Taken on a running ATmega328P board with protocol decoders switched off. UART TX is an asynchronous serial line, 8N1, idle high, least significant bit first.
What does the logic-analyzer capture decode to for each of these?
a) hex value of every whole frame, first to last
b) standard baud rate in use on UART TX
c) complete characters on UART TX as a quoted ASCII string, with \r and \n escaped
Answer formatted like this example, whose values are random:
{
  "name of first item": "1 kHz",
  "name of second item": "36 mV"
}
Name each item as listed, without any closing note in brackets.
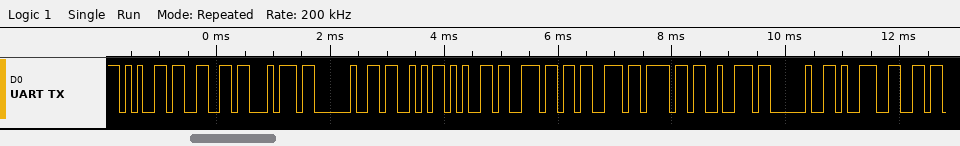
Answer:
{
  "hex value of every whole frame, first to last": "65 66 74 20 53 65 6E 73 6F 72 20 39",
  "standard baud rate in use on UART TX": "9600 baud",
  "complete characters on UART TX as a quoted ASCII string, with \\r and \\n escaped": "\"eft Sensor 9\""
}
